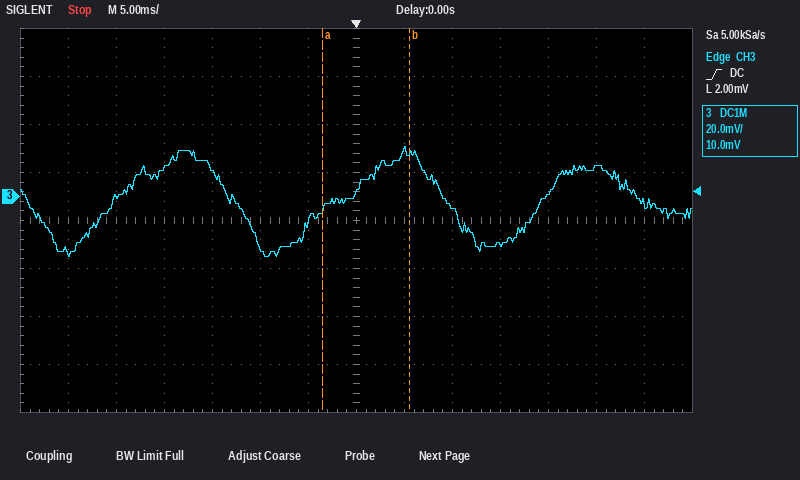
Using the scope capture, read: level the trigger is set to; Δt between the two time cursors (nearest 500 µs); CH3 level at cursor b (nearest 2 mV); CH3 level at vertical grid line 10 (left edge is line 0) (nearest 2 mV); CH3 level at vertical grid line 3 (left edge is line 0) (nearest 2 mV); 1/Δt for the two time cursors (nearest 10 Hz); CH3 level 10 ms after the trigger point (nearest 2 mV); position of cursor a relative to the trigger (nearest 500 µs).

2.00 mV
9.0 ms
18 mV
-20 mV
12 mV
110 Hz
-4 mV
-3.5 ms
